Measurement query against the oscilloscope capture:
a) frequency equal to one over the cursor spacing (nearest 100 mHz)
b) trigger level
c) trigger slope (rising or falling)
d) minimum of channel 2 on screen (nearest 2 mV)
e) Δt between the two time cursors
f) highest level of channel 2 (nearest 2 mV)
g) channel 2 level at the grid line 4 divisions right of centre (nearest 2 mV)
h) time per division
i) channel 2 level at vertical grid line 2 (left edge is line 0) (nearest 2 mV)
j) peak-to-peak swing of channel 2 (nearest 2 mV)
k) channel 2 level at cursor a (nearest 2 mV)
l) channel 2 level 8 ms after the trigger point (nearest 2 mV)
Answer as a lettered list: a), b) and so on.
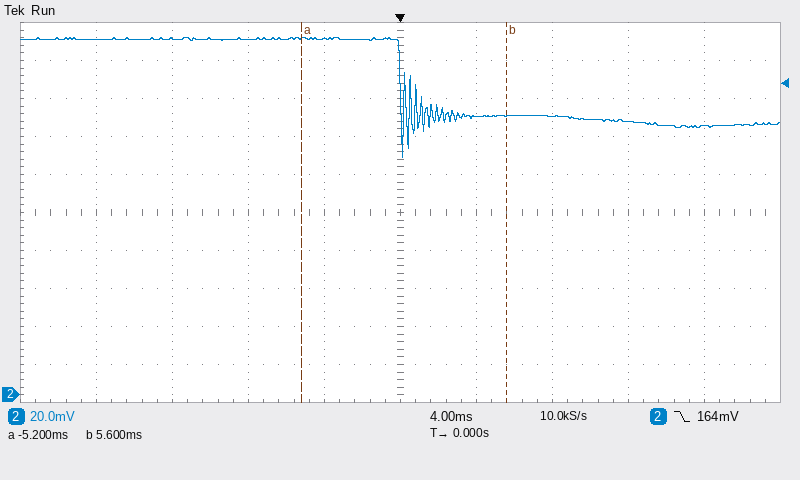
a) 92.6 Hz
b) 164 mV
c) falling
d) 124 mV
e) 10.8 ms
f) 188 mV
g) 142 mV
h) 4 ms
i) 188 mV
j) 64 mV
k) 188 mV
l) 146 mV
